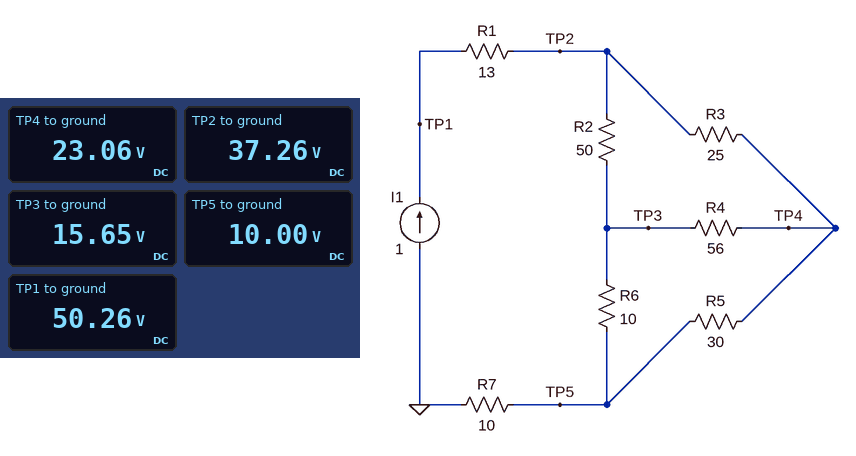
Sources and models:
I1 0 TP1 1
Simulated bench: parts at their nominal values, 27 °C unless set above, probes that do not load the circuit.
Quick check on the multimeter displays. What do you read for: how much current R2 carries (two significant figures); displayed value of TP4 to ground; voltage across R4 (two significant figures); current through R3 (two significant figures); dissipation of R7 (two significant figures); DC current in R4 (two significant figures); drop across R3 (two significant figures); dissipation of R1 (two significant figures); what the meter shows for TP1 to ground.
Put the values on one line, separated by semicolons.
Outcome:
430 mA; 23.06 V; 7.4 V; 570 mA; 10 W; 130 mA; 14 V; 13 W; 50.26 V
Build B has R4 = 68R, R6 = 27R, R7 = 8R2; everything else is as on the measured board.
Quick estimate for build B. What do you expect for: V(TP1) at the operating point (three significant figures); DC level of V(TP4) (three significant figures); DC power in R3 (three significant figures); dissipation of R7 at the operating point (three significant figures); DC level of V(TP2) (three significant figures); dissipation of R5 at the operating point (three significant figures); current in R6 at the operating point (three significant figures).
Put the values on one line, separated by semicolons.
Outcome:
52.9 V; 24.6 V; 9.31 W; 8.20 W; 39.9 V; 9.01 W; 452 mA
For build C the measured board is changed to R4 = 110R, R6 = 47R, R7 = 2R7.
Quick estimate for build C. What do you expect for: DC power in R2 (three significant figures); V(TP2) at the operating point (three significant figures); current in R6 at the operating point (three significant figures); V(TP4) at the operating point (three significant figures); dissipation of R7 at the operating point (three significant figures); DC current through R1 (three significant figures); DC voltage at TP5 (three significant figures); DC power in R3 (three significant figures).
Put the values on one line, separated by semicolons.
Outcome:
6.28 W; 37.8 V; 369 mA; 21.6 V; 2.70 W; 1.00 A; 2.70 V; 10.4 W
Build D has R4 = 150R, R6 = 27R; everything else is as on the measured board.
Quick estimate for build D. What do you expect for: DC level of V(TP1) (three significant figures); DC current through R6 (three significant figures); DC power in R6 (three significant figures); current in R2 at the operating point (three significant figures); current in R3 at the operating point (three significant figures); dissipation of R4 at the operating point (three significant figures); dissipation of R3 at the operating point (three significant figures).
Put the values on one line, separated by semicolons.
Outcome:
54.9 V; 436 mA; 5.14 W; 402 mA; 598 mA; 176 mW; 8.94 W
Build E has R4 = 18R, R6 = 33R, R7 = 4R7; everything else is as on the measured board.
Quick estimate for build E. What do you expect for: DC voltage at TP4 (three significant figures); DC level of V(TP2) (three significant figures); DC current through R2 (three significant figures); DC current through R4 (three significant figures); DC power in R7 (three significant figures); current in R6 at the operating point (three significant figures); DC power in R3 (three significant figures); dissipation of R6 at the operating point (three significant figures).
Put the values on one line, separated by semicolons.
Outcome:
21.2 V; 37.3 V; 356 mA; 93.6 mA; 4.70 W; 449 mA; 10.4 W; 6.67 W
